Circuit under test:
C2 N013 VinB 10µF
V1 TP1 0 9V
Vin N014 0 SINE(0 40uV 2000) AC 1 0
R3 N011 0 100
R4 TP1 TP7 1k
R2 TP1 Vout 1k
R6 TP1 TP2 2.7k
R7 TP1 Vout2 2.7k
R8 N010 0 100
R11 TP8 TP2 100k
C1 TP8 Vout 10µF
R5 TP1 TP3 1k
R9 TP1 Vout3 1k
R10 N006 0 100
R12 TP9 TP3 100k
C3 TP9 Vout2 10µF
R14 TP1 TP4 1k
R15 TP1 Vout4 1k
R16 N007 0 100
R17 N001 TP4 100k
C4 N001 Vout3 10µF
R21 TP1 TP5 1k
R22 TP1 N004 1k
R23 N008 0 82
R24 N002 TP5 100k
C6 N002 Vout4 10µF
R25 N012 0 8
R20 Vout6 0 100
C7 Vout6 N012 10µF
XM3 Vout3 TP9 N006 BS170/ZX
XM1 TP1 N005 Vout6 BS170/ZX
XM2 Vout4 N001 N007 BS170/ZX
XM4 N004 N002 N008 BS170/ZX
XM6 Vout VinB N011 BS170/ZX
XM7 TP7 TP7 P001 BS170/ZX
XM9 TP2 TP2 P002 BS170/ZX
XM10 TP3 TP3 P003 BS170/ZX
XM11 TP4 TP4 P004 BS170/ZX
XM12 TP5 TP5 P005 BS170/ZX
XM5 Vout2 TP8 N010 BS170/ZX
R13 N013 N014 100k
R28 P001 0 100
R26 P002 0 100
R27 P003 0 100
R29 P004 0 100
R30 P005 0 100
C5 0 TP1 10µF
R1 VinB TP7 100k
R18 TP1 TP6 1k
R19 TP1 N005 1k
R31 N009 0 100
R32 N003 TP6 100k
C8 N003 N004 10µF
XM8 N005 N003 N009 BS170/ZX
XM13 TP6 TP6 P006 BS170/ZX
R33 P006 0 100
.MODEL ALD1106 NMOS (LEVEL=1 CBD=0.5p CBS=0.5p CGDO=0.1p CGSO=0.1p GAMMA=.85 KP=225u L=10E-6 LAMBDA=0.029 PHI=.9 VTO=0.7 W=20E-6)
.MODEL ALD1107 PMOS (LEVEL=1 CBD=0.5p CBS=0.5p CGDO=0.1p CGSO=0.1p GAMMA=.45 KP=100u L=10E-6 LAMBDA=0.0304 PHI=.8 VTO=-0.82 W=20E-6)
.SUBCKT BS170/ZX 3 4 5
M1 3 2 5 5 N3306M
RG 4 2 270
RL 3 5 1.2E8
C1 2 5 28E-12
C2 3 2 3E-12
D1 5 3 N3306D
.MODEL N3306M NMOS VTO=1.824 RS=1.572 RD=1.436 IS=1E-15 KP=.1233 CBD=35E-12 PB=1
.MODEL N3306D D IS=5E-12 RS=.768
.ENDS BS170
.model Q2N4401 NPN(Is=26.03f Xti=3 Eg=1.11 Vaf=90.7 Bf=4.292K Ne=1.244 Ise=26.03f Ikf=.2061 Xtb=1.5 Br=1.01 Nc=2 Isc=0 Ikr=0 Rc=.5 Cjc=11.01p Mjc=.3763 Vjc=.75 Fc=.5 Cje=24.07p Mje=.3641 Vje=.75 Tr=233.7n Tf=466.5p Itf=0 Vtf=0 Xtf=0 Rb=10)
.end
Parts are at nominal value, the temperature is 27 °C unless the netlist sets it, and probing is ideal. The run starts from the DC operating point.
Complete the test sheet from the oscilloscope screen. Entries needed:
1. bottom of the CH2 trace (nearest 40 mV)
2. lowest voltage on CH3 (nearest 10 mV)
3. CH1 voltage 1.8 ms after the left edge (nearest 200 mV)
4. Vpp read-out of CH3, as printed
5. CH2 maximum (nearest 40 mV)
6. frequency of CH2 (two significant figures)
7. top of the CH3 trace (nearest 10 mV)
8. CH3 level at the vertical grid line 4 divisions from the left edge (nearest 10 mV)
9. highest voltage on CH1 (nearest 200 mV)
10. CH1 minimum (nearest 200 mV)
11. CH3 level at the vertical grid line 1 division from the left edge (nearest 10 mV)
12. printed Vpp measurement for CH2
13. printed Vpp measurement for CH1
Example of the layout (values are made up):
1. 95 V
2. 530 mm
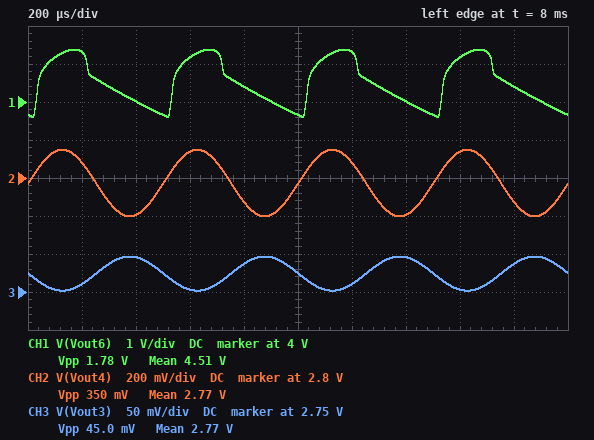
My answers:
1. 2.60 V
2. 2.75 V
3. 4.4 V
4. 45.0 mV
5. 2.96 V
6. 2.0 kHz
7. 2.80 V
8. 2.79 V
9. 5.4 V
10. 3.6 V
11. 2.76 V
12. 350 mV
13. 1.78 V
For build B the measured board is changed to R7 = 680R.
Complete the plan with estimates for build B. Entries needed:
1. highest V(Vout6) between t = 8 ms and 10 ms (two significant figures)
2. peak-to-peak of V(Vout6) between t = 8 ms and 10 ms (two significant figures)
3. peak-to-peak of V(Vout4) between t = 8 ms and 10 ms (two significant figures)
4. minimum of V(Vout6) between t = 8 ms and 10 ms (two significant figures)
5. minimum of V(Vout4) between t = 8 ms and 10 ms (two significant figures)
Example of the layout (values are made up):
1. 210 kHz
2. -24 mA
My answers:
1. 2.8 V
2. 1.1 V
3. 90 mV
4. 1.7 V
5. 2.7 V
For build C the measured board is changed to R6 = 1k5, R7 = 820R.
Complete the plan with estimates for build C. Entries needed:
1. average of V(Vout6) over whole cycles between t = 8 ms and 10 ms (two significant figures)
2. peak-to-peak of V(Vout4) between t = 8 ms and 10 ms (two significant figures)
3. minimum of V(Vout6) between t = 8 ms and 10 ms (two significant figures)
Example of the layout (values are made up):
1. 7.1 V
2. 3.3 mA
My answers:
1. 2.7 V
2. 120 mV
3. 2.1 V
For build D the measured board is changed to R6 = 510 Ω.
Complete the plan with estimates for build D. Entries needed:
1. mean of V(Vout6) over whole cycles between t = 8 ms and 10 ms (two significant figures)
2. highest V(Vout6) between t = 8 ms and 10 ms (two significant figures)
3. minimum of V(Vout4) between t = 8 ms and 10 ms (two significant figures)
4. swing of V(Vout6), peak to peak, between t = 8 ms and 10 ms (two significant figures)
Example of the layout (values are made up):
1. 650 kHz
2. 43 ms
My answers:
1. 620 mV
2. 630 mV
3. 2.8 V
4. 6.9 mV
